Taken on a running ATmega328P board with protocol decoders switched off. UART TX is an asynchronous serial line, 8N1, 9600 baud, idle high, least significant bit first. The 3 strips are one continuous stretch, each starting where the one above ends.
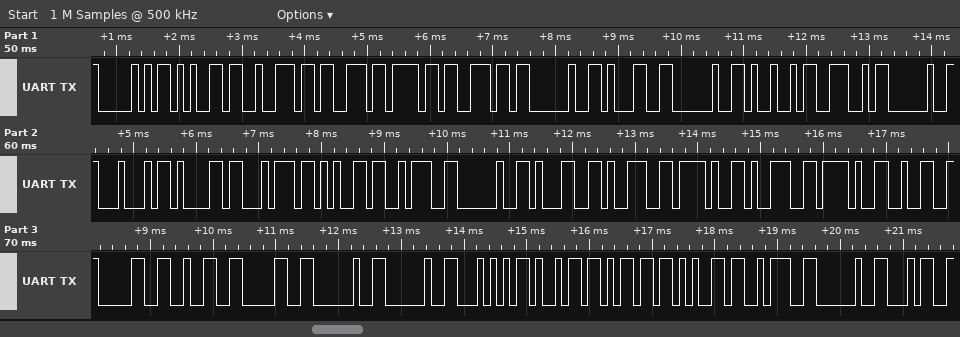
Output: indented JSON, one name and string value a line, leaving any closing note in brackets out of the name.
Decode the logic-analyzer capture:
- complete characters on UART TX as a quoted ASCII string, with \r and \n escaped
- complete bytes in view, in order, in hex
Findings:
{
  "complete characters on UART TX as a quoted ASCII string, with \\r and \\n escaped": "\"Person 1 IN Date: 19/9/2020  Time: 4\"",
  "complete bytes in view, in order, in hex": "50 65 72 73 6F 6E 20 31 20 49 4E 20 44 61 74 65 3A 20 31 39 2F 39 2F 32 30 32 30 20 20 54 69 6D 65 3A 20 34"
}
